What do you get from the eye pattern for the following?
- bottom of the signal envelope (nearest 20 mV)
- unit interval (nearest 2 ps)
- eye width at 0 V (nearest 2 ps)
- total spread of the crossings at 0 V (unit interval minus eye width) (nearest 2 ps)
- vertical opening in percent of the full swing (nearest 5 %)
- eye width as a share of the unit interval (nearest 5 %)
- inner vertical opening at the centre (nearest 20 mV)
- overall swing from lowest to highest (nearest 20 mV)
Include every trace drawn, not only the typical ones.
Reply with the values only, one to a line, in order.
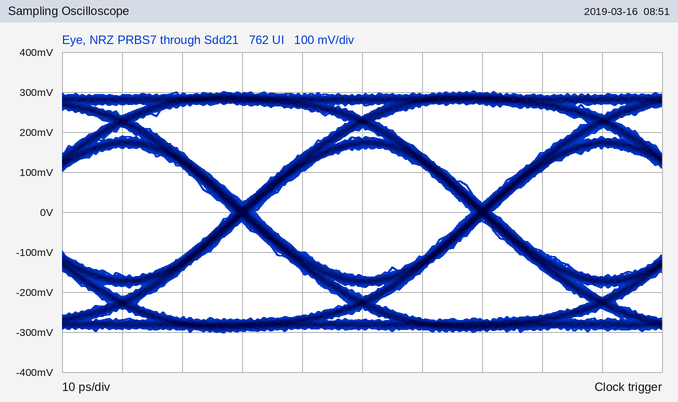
-300 mV
40 ps
36 ps
4 ps
55 %
90 %
320 mV
600 mV
